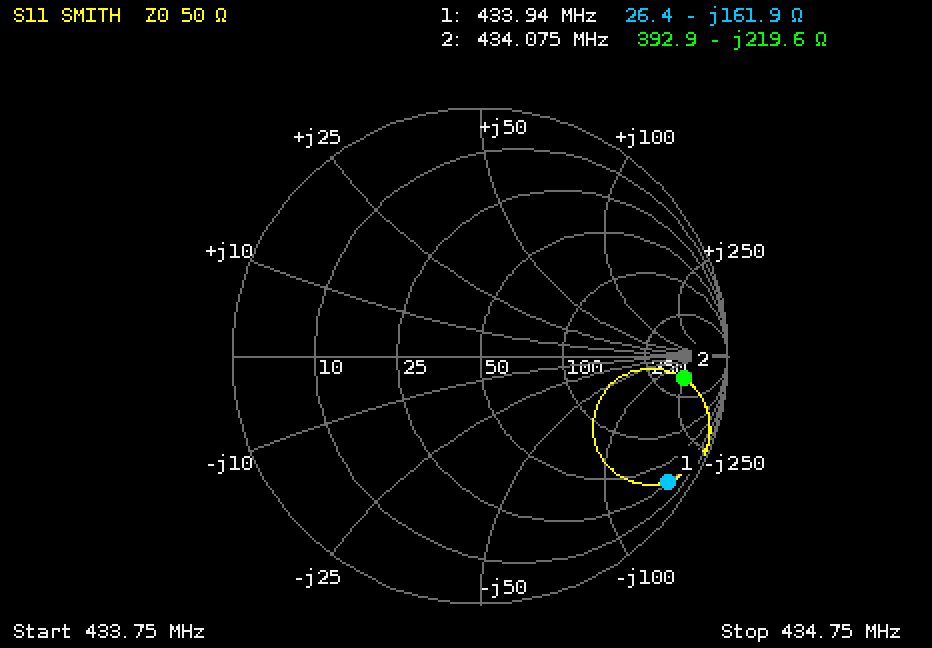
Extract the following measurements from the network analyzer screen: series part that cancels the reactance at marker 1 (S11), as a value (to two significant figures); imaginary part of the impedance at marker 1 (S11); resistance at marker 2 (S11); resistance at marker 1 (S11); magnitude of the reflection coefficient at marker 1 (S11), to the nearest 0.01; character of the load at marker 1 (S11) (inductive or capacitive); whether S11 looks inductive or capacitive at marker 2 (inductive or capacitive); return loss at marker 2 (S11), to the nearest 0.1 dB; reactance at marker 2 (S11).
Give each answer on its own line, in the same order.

59 nH
-161.9 Ω
392.9 Ω
26.4 Ω
0.91
capacitive
capacitive
1.7 dB
-219.6 Ω
